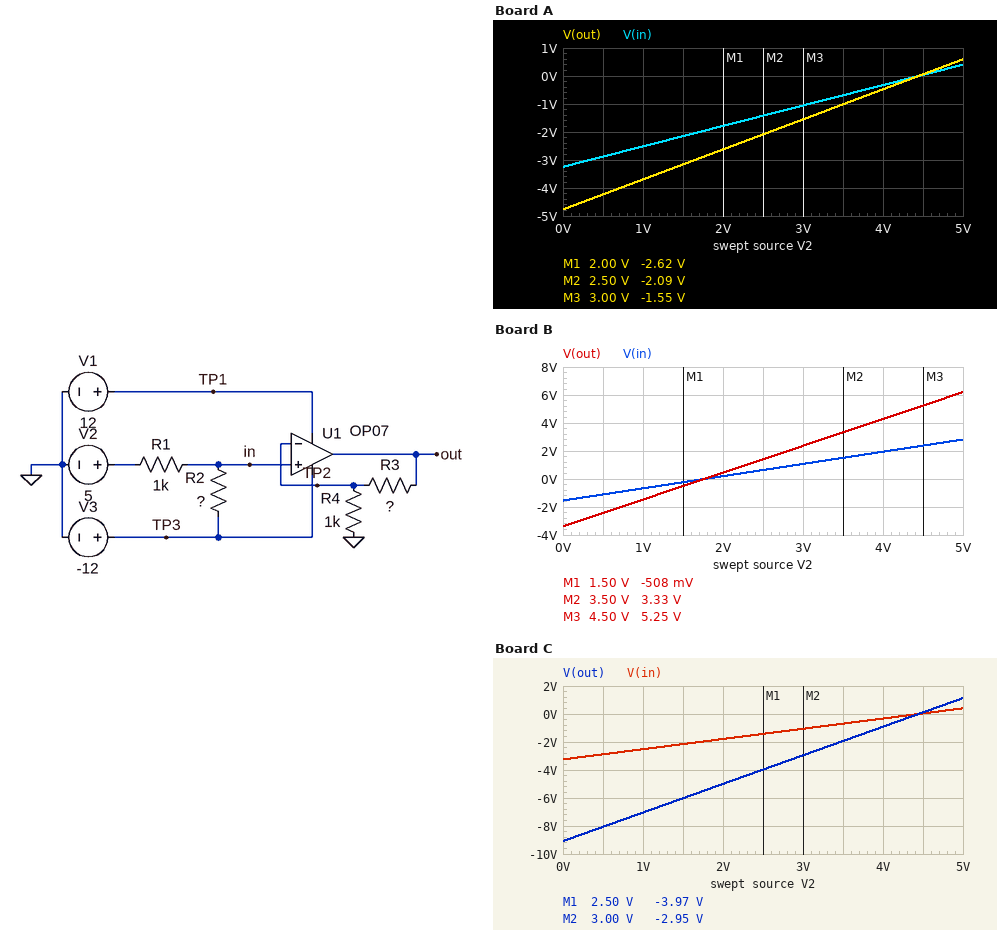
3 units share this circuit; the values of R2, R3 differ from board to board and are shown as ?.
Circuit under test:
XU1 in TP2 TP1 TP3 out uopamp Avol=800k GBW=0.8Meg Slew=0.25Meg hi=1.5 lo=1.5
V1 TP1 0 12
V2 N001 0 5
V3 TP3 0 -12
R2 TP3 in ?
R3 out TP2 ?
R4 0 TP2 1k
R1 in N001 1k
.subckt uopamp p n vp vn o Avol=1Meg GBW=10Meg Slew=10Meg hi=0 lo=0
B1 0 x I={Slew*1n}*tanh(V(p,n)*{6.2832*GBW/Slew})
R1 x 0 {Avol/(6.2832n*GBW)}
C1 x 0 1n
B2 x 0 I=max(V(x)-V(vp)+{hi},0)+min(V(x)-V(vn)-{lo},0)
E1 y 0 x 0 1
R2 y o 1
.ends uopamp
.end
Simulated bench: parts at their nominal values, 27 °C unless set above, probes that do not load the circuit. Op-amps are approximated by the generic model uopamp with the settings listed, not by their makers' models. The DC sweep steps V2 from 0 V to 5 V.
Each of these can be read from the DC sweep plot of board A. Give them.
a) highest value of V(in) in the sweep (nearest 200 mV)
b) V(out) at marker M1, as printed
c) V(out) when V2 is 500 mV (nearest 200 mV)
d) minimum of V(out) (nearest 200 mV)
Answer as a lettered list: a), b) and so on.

a) 400 mV
b) -2.62 V
c) -4.2 V
d) -4.8 V
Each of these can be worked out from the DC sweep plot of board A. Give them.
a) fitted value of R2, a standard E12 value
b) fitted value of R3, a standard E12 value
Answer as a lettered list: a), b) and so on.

a) 2.7 kΩ
b) 470 Ω
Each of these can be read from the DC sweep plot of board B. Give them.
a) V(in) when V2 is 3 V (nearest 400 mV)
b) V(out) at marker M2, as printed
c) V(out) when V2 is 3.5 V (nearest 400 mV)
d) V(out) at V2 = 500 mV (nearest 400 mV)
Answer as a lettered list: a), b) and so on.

a) 1.2 V
b) 3.33 V
c) 3.2 V
d) -2.4 V
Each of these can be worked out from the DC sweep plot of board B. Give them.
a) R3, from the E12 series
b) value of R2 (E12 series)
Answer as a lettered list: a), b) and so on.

a) 1.2 kΩ
b) 6.8 kΩ
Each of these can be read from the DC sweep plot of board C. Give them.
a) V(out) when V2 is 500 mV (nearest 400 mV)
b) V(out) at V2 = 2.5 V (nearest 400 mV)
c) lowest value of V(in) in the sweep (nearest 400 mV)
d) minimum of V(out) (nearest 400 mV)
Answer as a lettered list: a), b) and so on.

a) -8.0 V
b) -4.0 V
c) -3.2 V
d) -9.2 V
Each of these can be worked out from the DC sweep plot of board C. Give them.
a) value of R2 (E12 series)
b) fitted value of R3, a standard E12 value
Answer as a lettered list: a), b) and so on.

a) 2.7 kΩ
b) 1.8 kΩ
